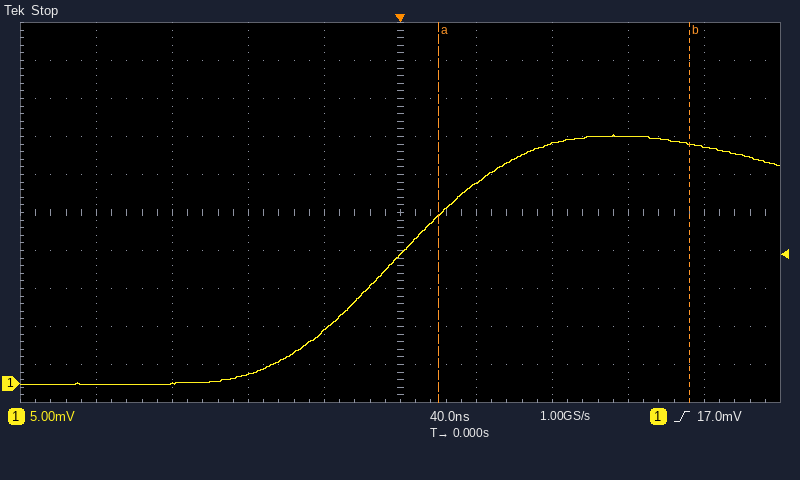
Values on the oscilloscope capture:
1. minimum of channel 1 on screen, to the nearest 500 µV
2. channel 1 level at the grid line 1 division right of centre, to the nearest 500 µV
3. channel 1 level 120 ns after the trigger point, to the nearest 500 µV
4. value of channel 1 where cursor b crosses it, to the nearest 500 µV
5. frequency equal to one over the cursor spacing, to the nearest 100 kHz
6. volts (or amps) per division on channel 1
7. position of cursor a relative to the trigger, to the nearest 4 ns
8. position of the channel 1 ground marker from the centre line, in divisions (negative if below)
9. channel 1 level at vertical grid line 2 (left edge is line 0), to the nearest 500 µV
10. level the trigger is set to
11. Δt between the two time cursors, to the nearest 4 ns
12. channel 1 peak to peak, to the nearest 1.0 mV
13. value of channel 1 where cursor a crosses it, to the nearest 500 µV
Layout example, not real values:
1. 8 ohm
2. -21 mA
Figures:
1. 0.0 mV
2. 26.5 mV
3. 32.5 mV
4. 31.5 mV
5. 7.6 MHz
6. 5 mV
7. +20 ns
8. -4.5 div
9. 0.0 mV
10. 17.0 mV
11. 132 ns
12. 33.0 mV
13. 22.0 mV
